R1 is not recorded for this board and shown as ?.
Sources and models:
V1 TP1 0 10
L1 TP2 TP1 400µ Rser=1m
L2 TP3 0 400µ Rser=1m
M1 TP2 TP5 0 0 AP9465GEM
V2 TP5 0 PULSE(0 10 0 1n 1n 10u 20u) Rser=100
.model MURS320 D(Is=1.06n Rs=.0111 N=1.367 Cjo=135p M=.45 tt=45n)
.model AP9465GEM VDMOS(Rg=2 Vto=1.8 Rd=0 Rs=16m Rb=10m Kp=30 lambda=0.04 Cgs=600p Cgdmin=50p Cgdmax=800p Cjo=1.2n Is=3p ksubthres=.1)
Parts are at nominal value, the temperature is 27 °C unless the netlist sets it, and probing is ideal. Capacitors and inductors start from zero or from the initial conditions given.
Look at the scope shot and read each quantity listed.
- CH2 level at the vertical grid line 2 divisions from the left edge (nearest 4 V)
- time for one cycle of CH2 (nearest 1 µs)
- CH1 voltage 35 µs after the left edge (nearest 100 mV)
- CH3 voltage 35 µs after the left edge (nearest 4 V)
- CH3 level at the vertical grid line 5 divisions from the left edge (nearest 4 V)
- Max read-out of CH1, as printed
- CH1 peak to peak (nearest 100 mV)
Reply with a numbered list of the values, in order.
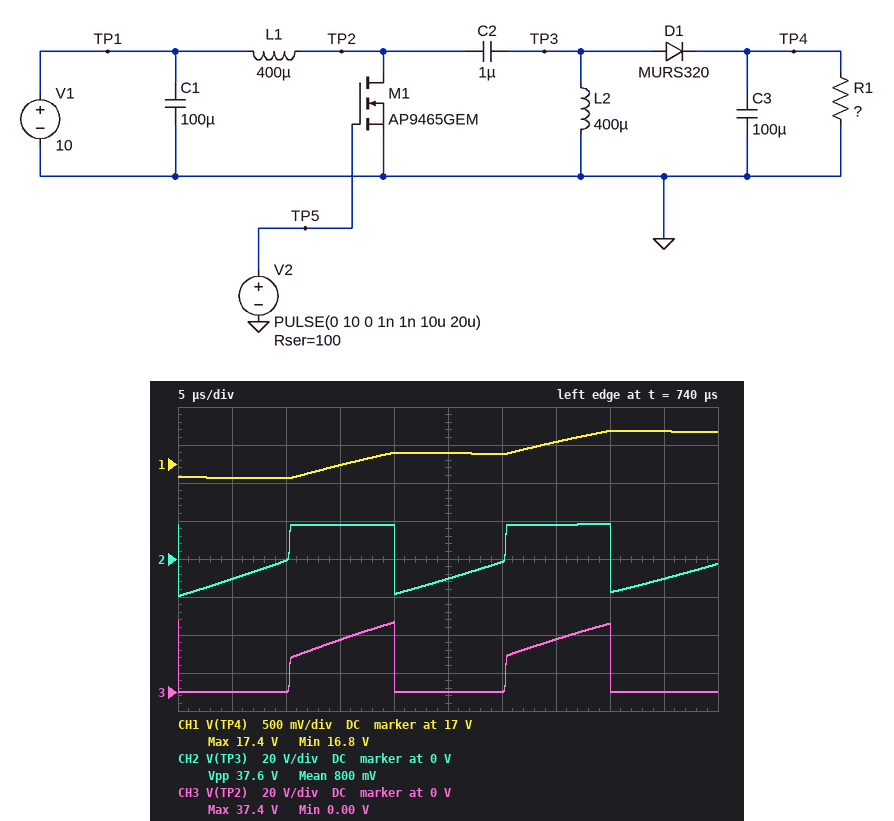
1. 0 V
2. 20 µs
3. 17.3 V
4. 28 V
5. 0 V
6. 17.4 V
7. 600 mV
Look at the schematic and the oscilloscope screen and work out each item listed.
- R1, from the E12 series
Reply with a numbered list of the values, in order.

1. 120 Ω
